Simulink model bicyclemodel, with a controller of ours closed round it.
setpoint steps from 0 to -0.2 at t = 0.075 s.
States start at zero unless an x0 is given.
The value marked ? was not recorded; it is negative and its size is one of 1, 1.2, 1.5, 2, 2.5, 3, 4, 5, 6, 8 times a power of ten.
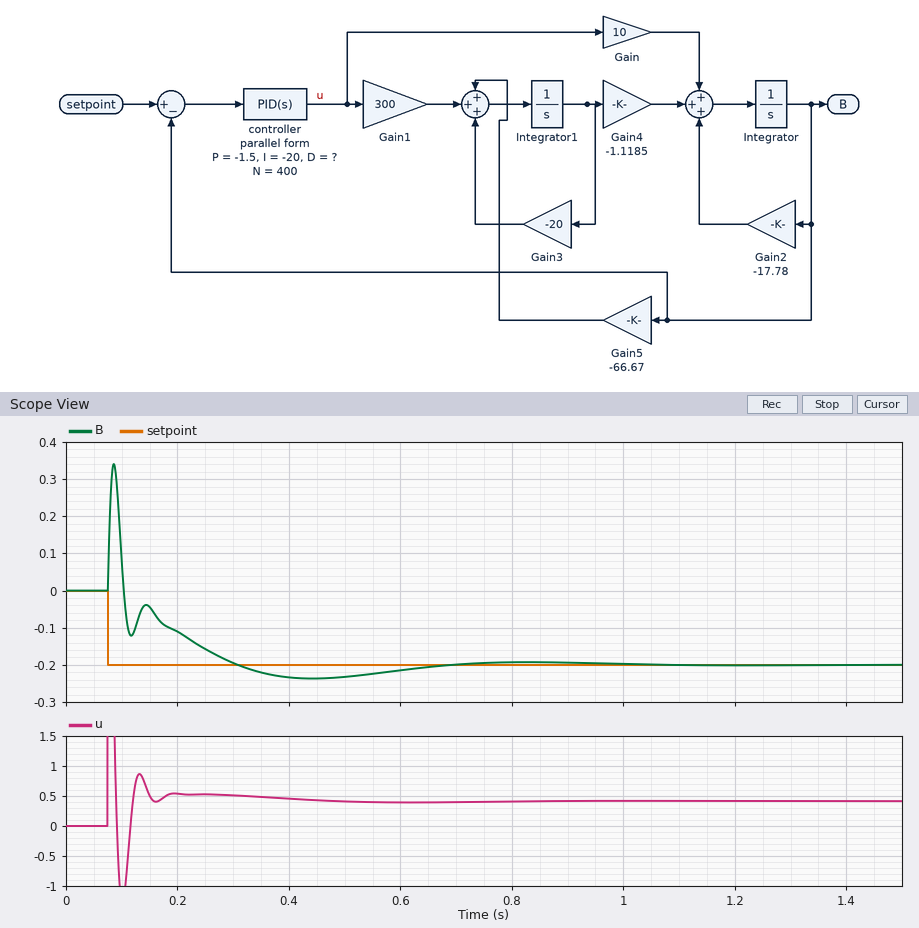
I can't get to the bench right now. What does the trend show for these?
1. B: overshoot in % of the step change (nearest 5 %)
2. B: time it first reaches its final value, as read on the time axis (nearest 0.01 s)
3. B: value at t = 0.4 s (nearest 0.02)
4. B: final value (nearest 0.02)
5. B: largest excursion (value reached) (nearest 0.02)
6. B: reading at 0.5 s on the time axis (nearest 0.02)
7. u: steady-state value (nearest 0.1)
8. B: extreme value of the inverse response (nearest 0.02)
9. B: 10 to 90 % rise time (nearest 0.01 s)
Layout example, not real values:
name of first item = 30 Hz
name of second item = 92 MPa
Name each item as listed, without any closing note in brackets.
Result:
B: overshoot in % of the step change = 20 %
B: time it first reaches its final value, as read on the time axis = 0.31 s
B: value at t = 0.4 s = -0.24
B: final value = -0.20
B: largest excursion (value reached) = -0.24
B: reading at 0.5 s on the time axis = -0.24
u: steady-state value = 0.4
B: extreme value of the inverse response = 0.34
B: 10 to 90 % rise time = 0.17 s
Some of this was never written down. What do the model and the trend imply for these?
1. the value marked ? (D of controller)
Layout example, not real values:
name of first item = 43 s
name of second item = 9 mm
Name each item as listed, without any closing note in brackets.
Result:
the value marked ? = -0.08
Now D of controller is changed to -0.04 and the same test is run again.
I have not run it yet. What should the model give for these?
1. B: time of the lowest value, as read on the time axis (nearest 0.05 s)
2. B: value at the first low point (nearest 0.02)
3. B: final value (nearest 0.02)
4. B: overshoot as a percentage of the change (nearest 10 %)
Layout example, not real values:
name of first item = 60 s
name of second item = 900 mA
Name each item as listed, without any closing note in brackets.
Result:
B: time of the lowest value, as read on the time axis = 0.40 s
B: value at the first low point = -0.26
B: final value = -0.20
B: overshoot as a percentage of the change = 30 %
